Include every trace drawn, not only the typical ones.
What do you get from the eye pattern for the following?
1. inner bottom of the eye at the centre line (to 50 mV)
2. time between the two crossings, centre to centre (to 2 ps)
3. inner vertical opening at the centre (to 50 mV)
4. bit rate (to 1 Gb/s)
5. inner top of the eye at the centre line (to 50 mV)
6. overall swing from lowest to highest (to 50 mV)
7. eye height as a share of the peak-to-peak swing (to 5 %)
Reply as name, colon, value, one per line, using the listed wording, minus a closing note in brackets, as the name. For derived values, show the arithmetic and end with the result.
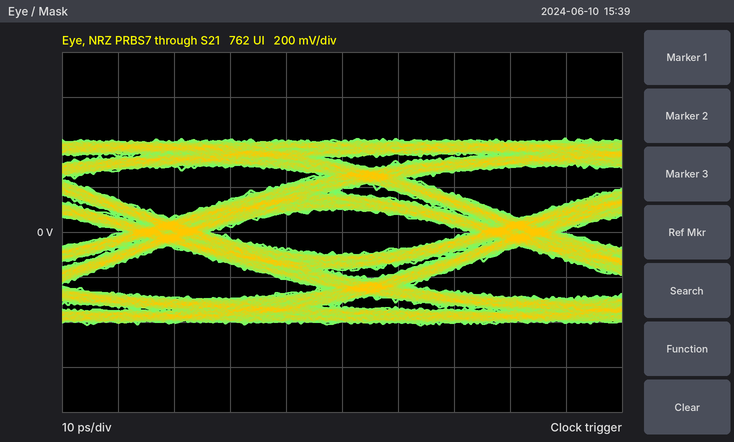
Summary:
inner bottom of the eye at the centre line: -100 mV
time between the two crossings, centre to centre: 62 ps
inner vertical opening at the centre: 200 mV
bit rate: 16 Gb/s
inner top of the eye at the centre line: 100 mV
overall swing from lowest to highest: 850 mV
eye height as a share of the peak-to-peak swing: 200 mV / 850 mV ≈ 23.5 %, so 25 % to the nearest 5 %
